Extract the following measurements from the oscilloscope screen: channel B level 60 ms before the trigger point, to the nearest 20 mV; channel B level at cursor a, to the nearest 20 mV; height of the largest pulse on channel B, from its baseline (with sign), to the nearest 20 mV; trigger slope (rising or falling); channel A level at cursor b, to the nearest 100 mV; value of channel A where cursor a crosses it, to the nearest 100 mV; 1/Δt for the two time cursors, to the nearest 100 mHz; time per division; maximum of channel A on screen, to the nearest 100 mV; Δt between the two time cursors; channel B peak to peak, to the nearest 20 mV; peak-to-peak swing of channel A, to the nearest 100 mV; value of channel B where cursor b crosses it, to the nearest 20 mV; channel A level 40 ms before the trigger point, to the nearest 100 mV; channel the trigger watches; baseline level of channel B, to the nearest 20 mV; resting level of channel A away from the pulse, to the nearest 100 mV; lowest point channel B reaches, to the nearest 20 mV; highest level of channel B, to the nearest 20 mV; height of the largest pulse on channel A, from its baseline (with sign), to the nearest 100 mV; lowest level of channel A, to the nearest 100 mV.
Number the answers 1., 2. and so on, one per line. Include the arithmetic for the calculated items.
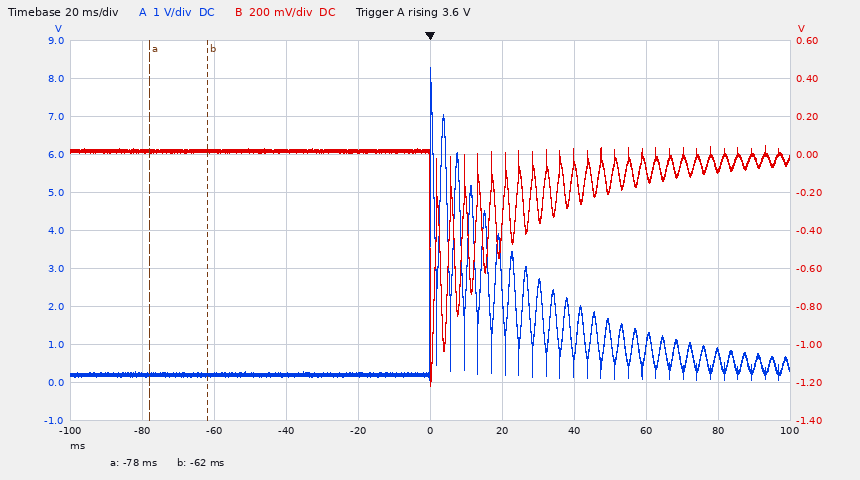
1. 20 mV
2. 20 mV
3. -1.22 V − (20 mV) = -1.24 V
4. rising
5. 200 mV
6. 200 mV
7. 1 / 16 ms ≈ 62.5 Hz
8. 20 ms
9. 8.3 V
10. -62 ms − (-78 ms) = 16 ms
11. 40 mV − (-1.22 V) = 1.26 V
12. 8.3 V − (100 mV) = 8.2 V
13. 20 mV
14. 200 mV
15. channel A
16. 20 mV
17. 200 mV
18. -1.22 V
19. 40 mV
20. 8.3 V − (200 mV) = +8.1 V
21. 100 mV
